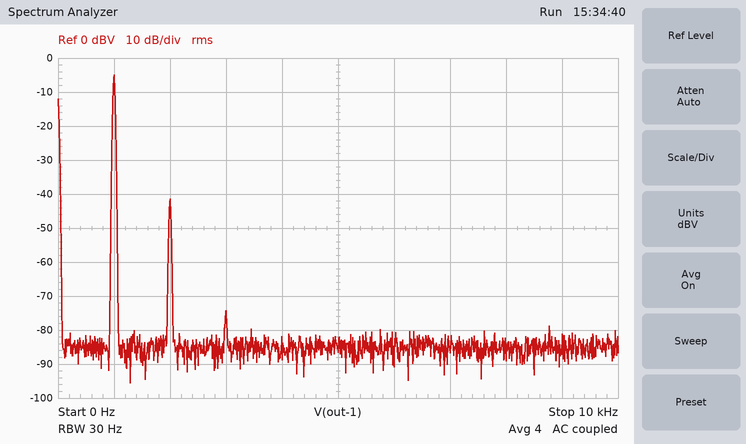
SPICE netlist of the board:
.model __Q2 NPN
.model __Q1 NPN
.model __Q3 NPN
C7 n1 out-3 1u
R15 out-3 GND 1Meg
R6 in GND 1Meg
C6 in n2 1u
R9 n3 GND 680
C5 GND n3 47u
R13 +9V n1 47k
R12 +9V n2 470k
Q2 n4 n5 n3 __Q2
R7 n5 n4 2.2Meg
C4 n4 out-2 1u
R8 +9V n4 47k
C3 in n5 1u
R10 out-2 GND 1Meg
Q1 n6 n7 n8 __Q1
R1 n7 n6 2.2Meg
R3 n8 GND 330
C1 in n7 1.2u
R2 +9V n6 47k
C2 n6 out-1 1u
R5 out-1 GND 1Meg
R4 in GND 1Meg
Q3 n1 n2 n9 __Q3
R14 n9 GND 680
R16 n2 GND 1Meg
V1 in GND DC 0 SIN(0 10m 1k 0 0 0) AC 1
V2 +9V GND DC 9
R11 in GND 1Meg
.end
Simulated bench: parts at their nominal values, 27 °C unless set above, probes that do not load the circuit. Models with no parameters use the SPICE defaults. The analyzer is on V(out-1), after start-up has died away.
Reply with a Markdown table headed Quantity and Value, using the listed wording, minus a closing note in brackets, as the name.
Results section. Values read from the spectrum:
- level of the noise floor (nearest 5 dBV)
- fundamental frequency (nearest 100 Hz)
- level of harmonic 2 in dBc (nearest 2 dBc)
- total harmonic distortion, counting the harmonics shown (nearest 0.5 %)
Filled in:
| Quantity | Value |
|---|---|
| level of the noise floor | -85 dBV |
| fundamental frequency | 1.0 kHz |
| level of harmonic 2 in dBc | -36 dBc |
| total harmonic distortion, counting the harmonics shown | 1.5 % |
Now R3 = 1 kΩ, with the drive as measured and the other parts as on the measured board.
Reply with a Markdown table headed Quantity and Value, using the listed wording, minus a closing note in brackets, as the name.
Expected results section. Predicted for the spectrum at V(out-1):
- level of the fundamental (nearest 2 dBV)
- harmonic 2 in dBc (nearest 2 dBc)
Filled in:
| Quantity | Value |
|---|---|
| level of the fundamental | -12 dBV |
| harmonic 2 in dBc | -50 dBc |
